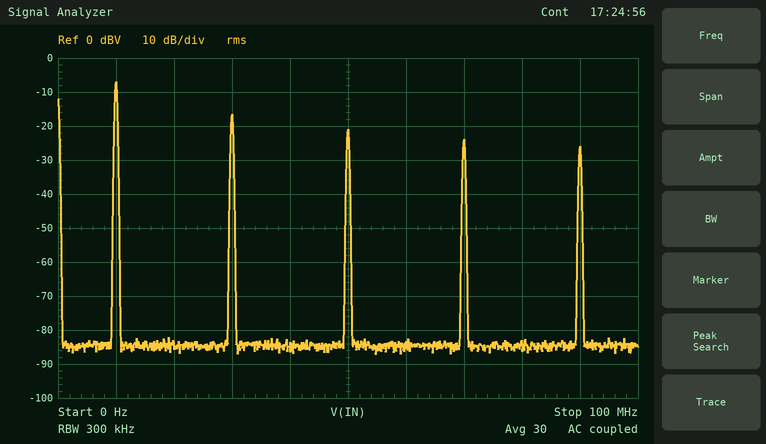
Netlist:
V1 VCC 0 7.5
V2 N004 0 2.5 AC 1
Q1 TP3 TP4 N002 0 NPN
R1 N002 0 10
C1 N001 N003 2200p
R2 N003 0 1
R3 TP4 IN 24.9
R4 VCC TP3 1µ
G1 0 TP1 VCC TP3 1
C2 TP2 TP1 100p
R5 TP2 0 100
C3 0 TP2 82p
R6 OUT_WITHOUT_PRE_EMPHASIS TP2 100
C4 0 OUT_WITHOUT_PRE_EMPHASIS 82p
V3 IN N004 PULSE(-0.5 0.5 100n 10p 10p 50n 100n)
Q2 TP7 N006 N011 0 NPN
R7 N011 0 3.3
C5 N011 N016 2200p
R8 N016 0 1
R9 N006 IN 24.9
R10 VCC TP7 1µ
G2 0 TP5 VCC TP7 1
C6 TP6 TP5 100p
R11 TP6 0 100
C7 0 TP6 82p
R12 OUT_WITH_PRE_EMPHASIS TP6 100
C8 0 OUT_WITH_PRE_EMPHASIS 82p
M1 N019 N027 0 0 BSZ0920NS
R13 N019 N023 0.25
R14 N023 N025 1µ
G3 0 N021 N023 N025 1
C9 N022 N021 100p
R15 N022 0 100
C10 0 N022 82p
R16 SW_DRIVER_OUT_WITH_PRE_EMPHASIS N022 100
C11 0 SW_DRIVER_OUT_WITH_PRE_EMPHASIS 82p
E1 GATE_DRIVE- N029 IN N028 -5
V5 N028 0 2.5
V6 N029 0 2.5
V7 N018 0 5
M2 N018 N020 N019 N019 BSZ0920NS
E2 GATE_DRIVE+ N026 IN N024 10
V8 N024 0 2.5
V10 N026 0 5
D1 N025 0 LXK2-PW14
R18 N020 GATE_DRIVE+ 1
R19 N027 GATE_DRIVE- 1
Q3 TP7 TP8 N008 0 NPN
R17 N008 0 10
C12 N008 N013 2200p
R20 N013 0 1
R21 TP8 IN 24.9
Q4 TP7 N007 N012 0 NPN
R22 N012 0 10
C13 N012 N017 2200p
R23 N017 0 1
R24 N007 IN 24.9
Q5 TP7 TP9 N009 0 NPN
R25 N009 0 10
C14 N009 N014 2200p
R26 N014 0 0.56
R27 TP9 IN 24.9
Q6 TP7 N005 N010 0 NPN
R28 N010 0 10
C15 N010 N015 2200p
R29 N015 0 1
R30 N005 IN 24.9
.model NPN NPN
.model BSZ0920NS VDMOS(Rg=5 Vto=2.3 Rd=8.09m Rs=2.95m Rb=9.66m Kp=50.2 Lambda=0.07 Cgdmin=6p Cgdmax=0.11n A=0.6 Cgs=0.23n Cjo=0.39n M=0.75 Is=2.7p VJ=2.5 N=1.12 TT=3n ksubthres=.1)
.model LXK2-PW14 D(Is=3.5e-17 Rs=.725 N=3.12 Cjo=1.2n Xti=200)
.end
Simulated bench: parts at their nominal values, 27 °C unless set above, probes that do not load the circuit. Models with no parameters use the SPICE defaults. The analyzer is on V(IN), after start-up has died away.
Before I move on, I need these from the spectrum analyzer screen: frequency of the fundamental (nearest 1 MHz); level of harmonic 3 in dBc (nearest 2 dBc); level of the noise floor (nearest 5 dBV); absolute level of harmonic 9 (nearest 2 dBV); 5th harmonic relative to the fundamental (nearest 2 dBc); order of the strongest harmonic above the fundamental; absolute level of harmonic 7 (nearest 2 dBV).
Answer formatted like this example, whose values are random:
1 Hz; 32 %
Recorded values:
10 MHz; -10 dBc; -85 dBV; -26 dBV; -14 dBc; 3; -24 dBV
